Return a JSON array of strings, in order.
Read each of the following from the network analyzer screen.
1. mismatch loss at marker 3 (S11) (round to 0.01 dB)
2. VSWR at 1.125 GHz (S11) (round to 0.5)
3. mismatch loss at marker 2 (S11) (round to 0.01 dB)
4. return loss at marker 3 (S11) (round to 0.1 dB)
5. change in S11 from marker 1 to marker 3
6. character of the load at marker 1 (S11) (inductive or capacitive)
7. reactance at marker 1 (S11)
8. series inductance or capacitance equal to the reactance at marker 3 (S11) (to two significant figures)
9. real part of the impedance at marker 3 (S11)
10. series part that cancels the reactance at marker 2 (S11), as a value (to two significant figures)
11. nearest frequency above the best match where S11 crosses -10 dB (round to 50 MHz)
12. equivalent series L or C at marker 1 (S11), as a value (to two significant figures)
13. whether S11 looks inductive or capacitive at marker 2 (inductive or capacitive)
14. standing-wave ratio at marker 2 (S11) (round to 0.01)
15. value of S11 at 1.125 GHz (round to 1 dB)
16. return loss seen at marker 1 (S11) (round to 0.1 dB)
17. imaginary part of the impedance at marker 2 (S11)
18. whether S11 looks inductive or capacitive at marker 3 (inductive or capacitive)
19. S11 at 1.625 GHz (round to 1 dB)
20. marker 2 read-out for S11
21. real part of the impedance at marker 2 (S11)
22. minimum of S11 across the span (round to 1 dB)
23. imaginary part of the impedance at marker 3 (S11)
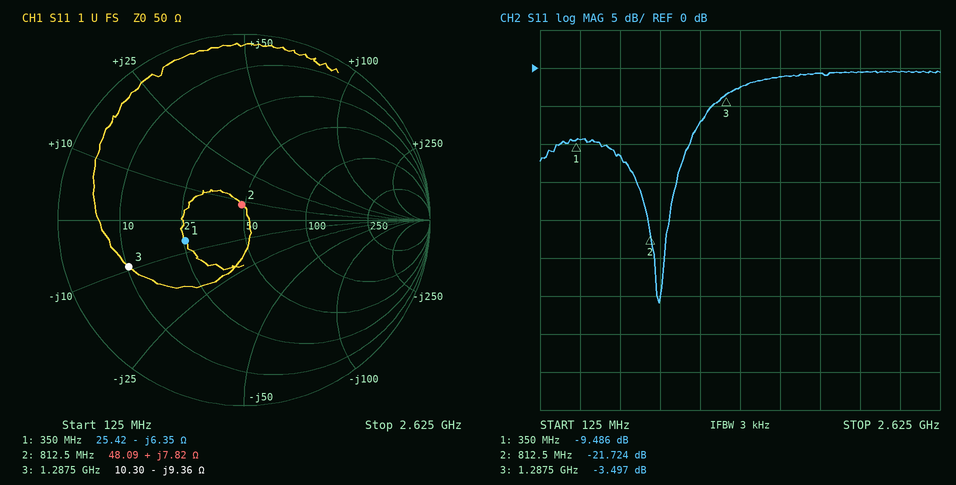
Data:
["2.57 dB", "2.5", "0.03 dB", "3.5 dB", "5.989 dB", "capacitive", "-6.35 Ω", "13 pF", "10.30 Ω", "25 pF", "1.05 GHz", "72 pF", "inductive", "1.18", "-7 dB", "9.5 dB", "+7.82 Ω", "capacitive", "-1 dB", "-21.724 dB", "48.09 Ω", "-31 dB", "-9.36 Ω"]
